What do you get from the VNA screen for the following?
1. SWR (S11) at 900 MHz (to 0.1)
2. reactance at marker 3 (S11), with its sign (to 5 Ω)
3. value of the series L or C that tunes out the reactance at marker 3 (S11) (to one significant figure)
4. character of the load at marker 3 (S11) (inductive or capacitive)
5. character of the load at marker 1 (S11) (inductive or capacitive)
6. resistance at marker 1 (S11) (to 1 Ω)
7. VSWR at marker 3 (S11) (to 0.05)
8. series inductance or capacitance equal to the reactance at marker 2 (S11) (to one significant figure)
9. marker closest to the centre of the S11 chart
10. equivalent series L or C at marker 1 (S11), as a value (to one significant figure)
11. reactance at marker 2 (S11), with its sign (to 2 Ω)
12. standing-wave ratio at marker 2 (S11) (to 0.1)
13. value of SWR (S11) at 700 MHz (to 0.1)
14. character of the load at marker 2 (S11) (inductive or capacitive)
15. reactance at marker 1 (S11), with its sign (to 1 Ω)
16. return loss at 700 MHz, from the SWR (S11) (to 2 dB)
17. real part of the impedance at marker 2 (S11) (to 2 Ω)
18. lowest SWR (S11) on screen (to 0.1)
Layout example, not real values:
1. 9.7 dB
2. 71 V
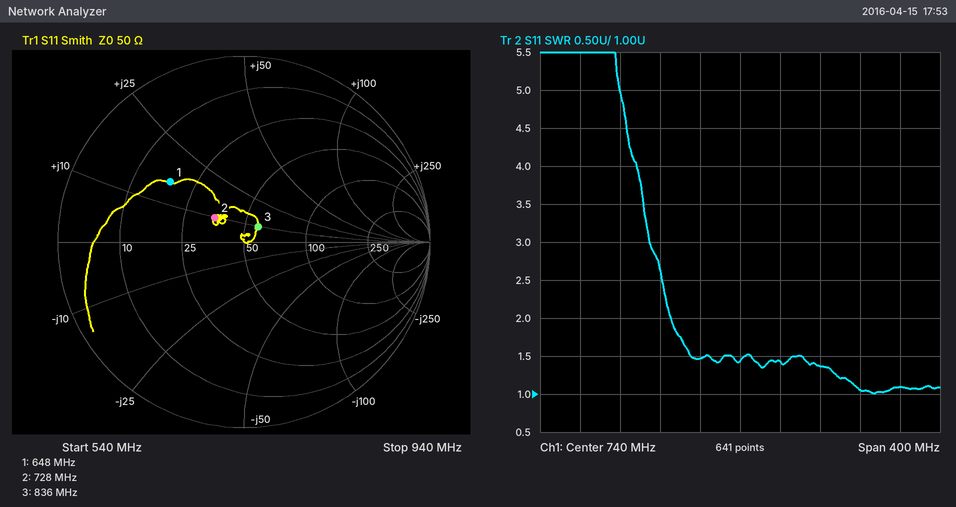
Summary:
1. 1.1
2. +10 Ω
3. 20 pF
4. inductive
5. inductive
6. 18 Ω
7. 1.25
8. 2 nH
9. marker 3
10. 4 nH
11. +10 Ω
12. 1.5
13. 1.5
14. inductive
15. +16 Ω
16. 14 dB
17. 36 Ω
18. 1.0
